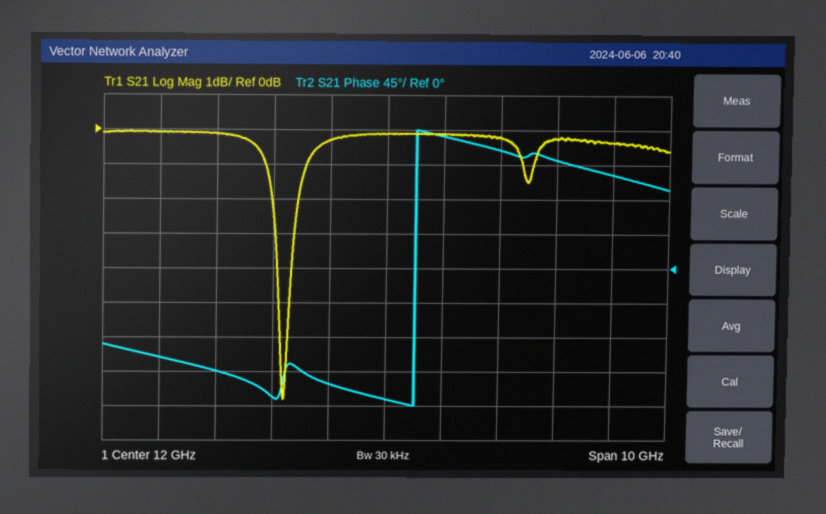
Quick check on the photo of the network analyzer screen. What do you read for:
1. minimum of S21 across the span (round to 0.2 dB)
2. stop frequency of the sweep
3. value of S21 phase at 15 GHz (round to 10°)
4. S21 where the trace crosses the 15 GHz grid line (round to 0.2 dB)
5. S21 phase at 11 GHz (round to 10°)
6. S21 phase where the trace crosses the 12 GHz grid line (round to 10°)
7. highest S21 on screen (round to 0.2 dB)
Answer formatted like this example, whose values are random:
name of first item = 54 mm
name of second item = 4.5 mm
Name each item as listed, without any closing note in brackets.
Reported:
minimum of S21 across the span = -7.8 dB
stop frequency of the sweep = 17 GHz
value of S21 phase at 15 GHz = 140°
S21 where the trace crosses the 15 GHz grid line = -0.2 dB
S21 phase at 11 GHz = -150°
S21 phase where the trace crosses the 12 GHz grid line = -170°
highest S21 on screen = 0.0 dB
